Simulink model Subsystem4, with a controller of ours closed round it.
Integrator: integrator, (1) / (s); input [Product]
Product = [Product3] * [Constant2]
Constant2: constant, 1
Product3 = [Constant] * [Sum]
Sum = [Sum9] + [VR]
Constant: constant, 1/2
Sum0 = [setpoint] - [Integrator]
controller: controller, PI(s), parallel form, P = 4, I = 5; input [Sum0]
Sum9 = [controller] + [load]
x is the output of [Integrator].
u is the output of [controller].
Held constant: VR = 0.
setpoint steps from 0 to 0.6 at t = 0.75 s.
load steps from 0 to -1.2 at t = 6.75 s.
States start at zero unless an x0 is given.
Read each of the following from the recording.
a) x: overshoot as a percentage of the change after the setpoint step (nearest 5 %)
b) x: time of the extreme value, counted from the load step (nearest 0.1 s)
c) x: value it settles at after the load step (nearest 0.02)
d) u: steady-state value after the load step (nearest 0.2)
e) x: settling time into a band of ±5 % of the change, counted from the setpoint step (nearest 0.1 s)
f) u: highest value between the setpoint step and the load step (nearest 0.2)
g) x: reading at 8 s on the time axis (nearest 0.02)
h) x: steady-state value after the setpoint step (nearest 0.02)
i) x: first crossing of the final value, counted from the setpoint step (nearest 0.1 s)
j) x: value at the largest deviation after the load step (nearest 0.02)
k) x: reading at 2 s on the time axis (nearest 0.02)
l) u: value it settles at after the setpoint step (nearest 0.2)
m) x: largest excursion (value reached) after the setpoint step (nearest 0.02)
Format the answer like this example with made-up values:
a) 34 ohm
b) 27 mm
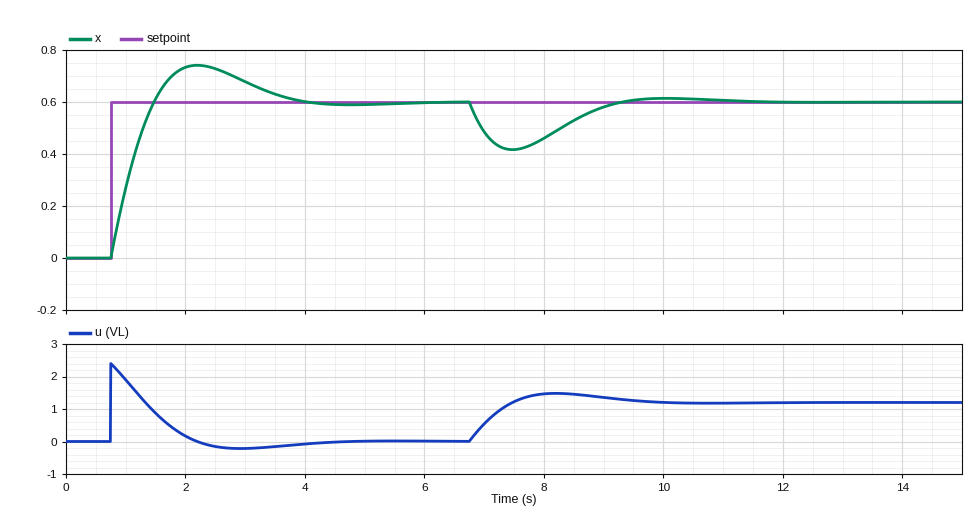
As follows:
a) 25 %
b) 0.7 s
c) 0.60
d) 1.2
e) 2.8 s
f) 2.4
g) 0.46
h) 0.60
i) 0.7 s
j) 0.42
k) 0.74
l) 0.0
m) 0.74
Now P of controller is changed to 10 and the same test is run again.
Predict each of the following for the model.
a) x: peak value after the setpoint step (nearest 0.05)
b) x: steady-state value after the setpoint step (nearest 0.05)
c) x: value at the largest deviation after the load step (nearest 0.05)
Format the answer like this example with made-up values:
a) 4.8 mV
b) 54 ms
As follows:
a) 0.65
b) 0.60
c) 0.50
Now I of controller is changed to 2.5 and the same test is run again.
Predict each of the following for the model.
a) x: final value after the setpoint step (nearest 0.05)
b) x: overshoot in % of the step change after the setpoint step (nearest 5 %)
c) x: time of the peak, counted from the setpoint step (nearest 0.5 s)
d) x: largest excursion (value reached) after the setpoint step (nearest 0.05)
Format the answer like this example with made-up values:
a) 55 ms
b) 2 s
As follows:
a) 0.60
b) 15 %
c) 2.0 s
d) 0.70
